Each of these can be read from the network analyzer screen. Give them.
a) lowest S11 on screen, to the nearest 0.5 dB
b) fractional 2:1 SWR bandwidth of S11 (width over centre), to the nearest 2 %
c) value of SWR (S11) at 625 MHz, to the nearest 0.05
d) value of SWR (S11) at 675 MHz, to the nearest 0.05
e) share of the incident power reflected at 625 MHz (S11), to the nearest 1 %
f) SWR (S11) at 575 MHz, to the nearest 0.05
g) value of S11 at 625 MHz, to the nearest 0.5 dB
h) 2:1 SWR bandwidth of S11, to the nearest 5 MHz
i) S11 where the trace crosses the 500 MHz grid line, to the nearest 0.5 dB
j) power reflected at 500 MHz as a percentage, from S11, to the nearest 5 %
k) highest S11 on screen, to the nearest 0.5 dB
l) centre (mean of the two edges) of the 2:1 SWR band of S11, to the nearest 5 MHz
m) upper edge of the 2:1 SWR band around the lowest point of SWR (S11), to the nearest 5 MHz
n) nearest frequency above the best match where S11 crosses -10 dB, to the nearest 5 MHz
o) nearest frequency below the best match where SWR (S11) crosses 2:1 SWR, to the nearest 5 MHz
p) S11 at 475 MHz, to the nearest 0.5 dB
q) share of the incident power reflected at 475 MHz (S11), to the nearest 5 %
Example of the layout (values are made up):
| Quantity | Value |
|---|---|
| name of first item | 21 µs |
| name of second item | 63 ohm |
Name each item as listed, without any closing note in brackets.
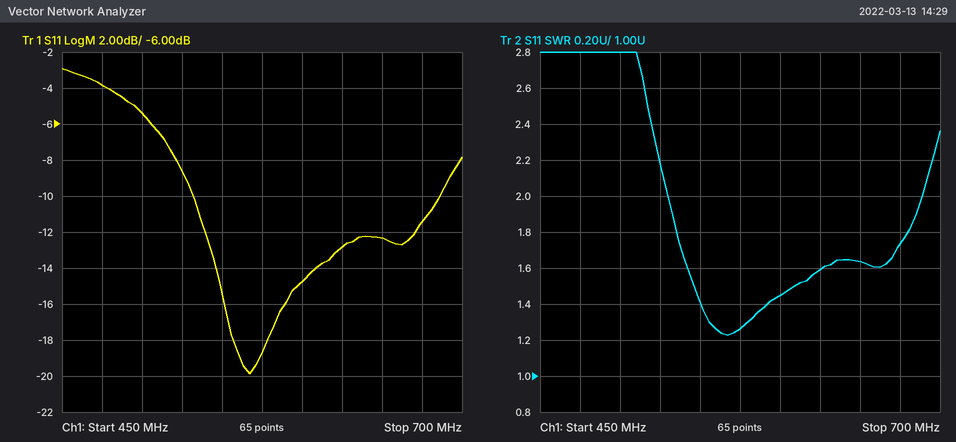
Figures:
| Quantity | Value |
|---|---|
| lowest S11 on screen, to the nearest 0.5 dB | -20.0 dB |
| fractional 2:1 SWR bandwidth of S11 (width over centre), to the nearest 2 % | 26 % |
| value of SWR (S11) at 625 MHz, to the nearest 0.05 | 1.60 |
| value of SWR (S11) at 675 MHz, to the nearest 0.05 | 1.75 |
| share of the incident power reflected at 625 MHz (S11), to the nearest 1 % | 5 % |
| SWR (S11) at 575 MHz, to the nearest 0.05 | 1.25 |
| value of S11 at 625 MHz, to the nearest 0.5 dB | -13.0 dB |
| 2:1 SWR bandwidth of S11, to the nearest 5 MHz | 160 MHz |
| S11 where the trace crosses the 500 MHz grid line, to the nearest 0.5 dB | -5.5 dB |
| power reflected at 500 MHz as a percentage, from S11, to the nearest 5 % | 30 % |
| highest S11 on screen, to the nearest 0.5 dB | -3.0 dB |
| centre (mean of the two edges) of the 2:1 SWR band of S11, to the nearest 5 MHz | 610 MHz |
| upper edge of the 2:1 SWR band around the lowest point of SWR (S11), to the nearest 5 MHz | 690 MHz |
| nearest frequency above the best match where S11 crosses -10 dB, to the nearest 5 MHz | 685 MHz |
| nearest frequency below the best match where SWR (S11) crosses 2:1 SWR, to the nearest 5 MHz | 530 MHz |
| S11 at 475 MHz, to the nearest 0.5 dB | -4.0 dB |
| share of the incident power reflected at 475 MHz (S11), to the nearest 5 % | 40 % |
